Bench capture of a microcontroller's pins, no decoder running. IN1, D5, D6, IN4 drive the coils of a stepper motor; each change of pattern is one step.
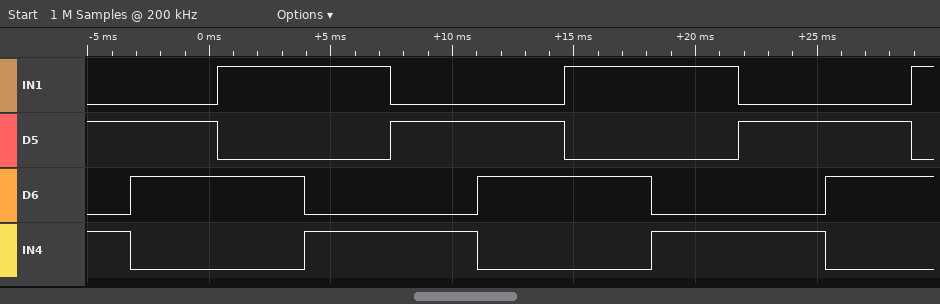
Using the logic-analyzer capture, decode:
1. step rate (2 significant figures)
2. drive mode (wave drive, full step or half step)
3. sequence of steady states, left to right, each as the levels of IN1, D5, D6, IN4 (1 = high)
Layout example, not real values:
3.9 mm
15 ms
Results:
280 steps/s
full step
0101 0110 1010 1001 0101 0110 1010 1001 0101 0110 1010
